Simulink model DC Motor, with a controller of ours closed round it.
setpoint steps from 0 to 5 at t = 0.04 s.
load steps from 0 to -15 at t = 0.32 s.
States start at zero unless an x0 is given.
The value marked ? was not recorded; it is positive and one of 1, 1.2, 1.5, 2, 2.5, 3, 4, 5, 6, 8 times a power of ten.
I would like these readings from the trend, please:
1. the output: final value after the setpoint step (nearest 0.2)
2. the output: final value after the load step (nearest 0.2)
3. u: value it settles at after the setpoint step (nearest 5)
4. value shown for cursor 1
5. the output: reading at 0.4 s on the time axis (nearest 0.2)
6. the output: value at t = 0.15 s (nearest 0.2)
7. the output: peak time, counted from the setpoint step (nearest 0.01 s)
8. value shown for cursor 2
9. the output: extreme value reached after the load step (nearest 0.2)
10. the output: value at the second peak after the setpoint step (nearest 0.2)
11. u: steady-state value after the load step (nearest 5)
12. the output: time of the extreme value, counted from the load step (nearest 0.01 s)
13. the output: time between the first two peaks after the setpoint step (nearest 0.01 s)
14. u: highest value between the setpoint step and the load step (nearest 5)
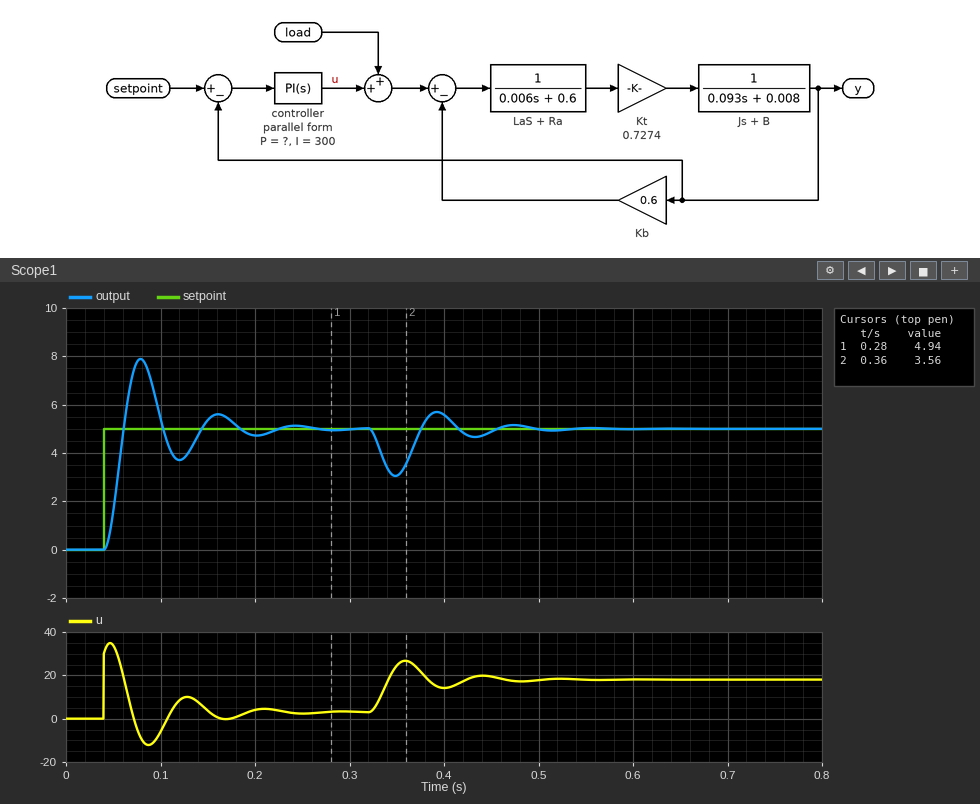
5.0
5.0
5
4.94
5.6
5.4
0.04 s
3.56
3.0
5.6
20
0.03 s
0.08 s
35
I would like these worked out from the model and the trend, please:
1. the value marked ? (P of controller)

6
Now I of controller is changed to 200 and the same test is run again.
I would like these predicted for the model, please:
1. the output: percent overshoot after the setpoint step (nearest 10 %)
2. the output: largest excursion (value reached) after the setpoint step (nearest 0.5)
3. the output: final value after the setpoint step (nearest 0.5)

40 %
7.0
5.0
